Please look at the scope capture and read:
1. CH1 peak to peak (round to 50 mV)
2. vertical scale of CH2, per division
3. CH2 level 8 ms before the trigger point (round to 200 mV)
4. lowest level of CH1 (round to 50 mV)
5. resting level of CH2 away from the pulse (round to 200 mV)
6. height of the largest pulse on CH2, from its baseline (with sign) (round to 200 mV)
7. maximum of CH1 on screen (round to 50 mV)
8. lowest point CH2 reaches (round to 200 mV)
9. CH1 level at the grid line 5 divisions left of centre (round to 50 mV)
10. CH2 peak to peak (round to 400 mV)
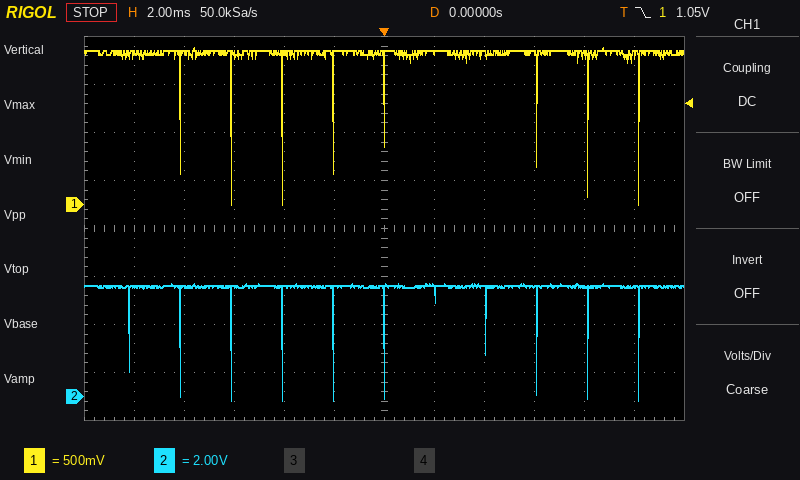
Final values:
1.65 V
2 V
4.6 V
0 mV
4.6 V
-4.8 V
1.65 V
-200 mV
1.55 V
4.8 V
